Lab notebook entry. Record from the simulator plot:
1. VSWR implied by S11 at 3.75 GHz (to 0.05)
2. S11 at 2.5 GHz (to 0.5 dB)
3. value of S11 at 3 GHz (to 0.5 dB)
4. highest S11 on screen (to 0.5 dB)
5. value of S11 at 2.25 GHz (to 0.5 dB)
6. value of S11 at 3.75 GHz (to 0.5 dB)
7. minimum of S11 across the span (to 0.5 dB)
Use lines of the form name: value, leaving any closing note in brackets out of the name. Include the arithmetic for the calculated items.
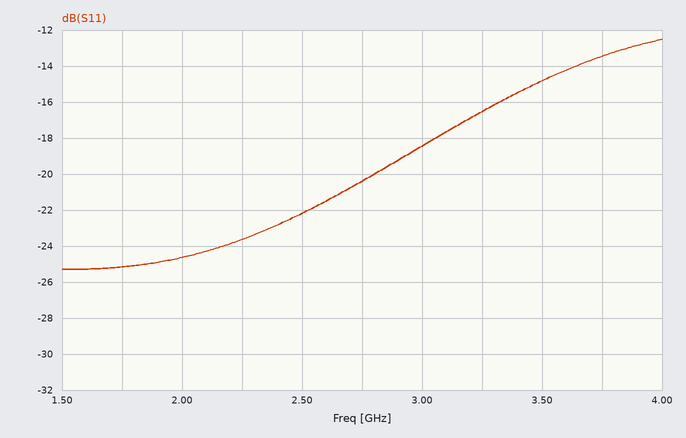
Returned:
VSWR implied by S11 at 3.75 GHz: |Γ| = 10^(-13.5/20) = 0.2113; VSWR = (1 + 0.2113)/(1 − 0.2113) ≈ 1.54, so 1.55 to the nearest 0.05
S11 at 2.5 GHz: -22.0 dB
value of S11 at 3 GHz: -18.5 dB
highest S11 on screen: -12.5 dB
value of S11 at 2.25 GHz: -23.5 dB
value of S11 at 3.75 GHz: -13.5 dB
minimum of S11 across the span: -25.5 dB
